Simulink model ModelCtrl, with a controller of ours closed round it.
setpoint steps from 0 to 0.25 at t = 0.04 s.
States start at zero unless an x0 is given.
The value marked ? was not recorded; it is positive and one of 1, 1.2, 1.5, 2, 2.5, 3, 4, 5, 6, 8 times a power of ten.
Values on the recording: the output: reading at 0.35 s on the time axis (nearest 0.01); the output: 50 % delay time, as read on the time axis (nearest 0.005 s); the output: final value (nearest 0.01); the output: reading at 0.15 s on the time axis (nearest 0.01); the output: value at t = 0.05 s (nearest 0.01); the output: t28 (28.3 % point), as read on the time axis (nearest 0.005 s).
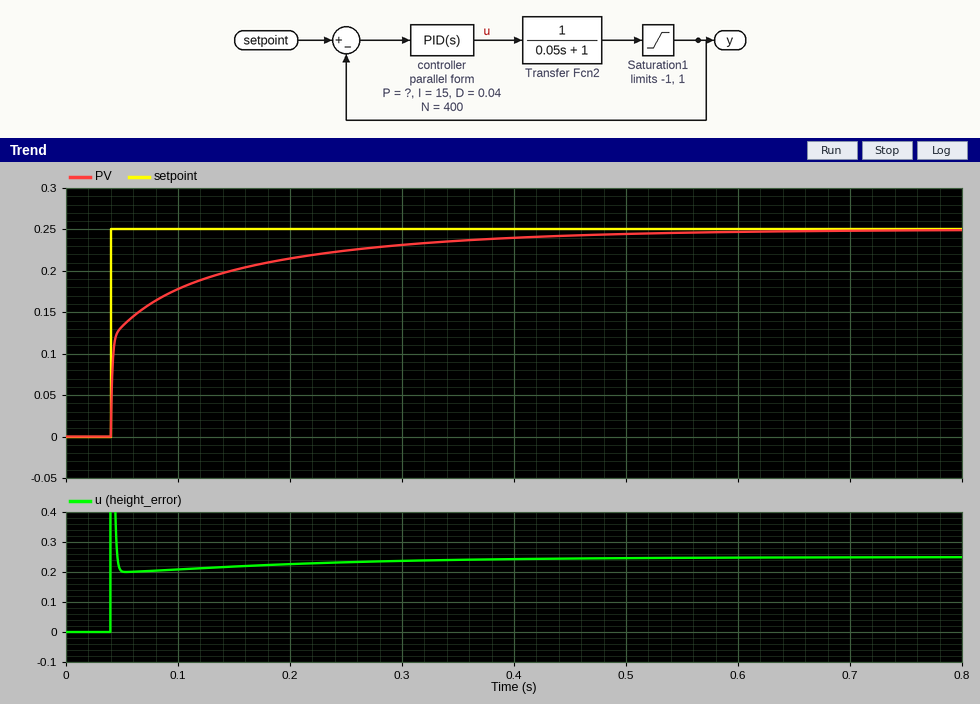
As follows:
0.24
0.045 s
0.25
0.20
0.13
0.040 s
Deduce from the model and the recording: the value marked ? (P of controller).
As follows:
2
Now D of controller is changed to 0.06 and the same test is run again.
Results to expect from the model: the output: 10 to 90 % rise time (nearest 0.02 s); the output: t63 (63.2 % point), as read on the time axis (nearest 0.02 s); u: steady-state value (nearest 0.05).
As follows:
0.22 s
0.06 s
0.25
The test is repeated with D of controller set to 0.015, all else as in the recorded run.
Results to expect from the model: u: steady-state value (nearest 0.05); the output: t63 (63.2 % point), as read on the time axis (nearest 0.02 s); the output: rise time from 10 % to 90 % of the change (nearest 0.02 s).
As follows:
0.25
0.08 s
0.20 s
